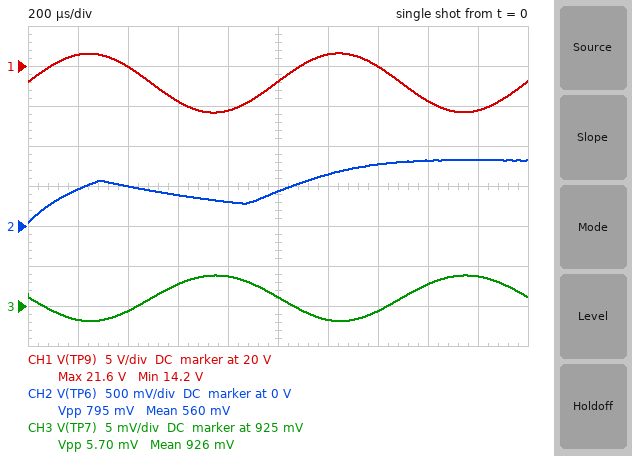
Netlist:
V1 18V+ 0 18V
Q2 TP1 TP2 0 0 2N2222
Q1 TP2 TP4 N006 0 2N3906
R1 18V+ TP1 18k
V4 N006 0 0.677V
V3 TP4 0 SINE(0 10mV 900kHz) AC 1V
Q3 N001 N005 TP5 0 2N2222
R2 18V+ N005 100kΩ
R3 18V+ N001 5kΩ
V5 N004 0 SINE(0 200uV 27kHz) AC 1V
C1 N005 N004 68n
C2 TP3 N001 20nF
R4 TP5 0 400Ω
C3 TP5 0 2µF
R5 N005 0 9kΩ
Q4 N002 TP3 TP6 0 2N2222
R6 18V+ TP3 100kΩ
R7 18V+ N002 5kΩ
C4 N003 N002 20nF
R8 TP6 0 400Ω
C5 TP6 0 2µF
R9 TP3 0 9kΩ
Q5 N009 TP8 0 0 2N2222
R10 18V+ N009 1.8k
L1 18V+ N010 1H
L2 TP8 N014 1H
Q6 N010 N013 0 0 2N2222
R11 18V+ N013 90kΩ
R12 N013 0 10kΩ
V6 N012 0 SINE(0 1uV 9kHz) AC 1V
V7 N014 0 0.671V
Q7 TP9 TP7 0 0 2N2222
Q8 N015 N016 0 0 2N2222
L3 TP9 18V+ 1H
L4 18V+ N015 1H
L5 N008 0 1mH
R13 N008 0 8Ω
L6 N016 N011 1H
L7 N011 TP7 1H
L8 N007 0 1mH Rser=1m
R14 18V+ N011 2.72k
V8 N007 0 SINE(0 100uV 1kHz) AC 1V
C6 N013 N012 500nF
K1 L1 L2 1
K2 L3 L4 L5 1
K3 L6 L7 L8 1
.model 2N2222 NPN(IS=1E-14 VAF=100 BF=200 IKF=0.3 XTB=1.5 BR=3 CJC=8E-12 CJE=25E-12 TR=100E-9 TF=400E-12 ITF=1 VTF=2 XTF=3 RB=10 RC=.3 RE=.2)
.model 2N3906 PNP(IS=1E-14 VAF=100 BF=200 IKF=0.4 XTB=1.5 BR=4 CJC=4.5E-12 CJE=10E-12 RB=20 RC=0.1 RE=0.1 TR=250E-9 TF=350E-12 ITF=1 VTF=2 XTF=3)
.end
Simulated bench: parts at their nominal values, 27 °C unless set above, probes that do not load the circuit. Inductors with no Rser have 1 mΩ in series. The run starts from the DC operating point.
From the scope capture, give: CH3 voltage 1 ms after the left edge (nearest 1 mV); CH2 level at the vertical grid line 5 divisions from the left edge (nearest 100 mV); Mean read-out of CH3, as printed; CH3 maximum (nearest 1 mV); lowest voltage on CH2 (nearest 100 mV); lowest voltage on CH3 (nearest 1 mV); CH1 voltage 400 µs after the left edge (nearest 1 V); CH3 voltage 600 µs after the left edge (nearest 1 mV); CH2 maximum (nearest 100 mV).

926 mV
400 mV
926 mV
929 mV
0 V
923 mV
20 V
928 mV
800 mV
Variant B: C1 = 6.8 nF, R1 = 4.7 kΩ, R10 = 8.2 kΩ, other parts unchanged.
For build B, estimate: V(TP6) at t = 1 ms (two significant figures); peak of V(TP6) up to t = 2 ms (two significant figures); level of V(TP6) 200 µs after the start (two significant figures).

870 mV
910 mV
88 mV
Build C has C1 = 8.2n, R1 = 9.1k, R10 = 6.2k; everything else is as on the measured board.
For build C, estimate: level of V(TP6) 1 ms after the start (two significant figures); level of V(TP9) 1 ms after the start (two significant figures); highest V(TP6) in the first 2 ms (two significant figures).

850 mV
18 V
910 mV
